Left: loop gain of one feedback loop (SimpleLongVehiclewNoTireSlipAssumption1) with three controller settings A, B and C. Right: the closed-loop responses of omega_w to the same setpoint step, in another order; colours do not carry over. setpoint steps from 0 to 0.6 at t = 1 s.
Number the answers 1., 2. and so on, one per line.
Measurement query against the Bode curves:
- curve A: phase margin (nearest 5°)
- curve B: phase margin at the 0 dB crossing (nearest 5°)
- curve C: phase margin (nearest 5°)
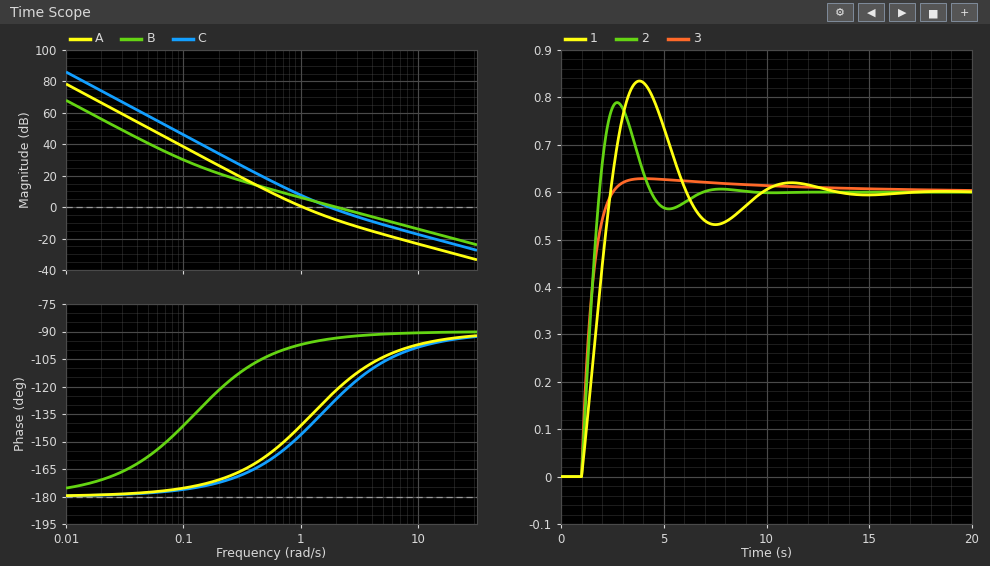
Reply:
1. 40°
2. 85°
3. 50°
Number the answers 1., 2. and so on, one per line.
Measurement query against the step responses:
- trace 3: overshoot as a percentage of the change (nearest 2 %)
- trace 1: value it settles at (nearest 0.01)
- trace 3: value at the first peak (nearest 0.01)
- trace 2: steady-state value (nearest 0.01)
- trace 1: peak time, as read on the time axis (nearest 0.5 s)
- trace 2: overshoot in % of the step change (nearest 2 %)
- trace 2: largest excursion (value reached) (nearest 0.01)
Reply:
1. 4 %
2. 0.60
3. 0.63
4. 0.60
5. 4.0 s
6. 32 %
7. 0.79
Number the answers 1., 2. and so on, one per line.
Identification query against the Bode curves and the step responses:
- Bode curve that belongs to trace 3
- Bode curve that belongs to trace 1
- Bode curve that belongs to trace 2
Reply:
1. B
2. A
3. C
